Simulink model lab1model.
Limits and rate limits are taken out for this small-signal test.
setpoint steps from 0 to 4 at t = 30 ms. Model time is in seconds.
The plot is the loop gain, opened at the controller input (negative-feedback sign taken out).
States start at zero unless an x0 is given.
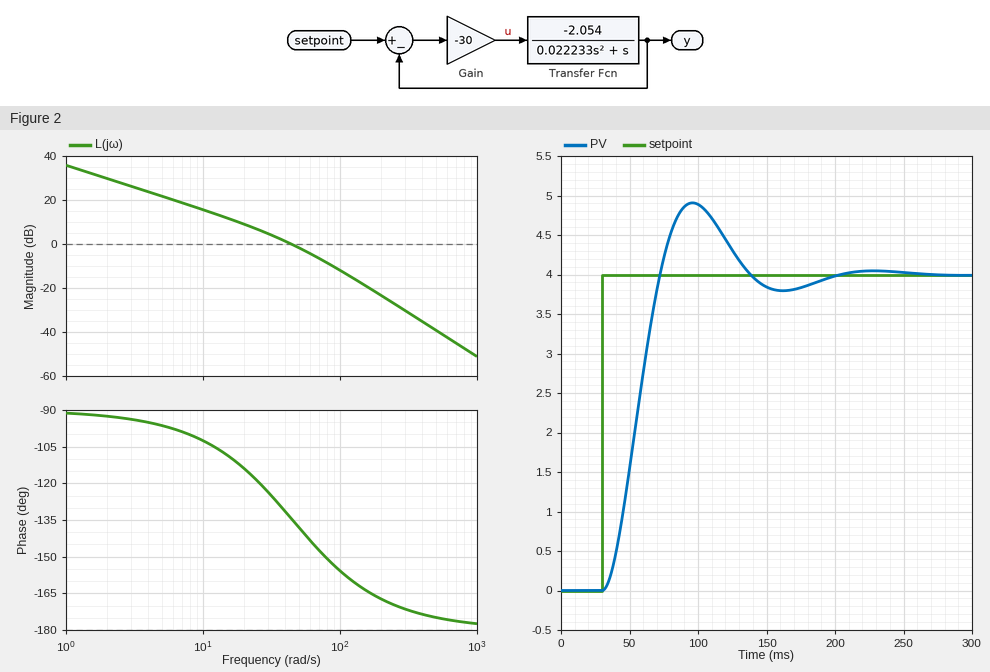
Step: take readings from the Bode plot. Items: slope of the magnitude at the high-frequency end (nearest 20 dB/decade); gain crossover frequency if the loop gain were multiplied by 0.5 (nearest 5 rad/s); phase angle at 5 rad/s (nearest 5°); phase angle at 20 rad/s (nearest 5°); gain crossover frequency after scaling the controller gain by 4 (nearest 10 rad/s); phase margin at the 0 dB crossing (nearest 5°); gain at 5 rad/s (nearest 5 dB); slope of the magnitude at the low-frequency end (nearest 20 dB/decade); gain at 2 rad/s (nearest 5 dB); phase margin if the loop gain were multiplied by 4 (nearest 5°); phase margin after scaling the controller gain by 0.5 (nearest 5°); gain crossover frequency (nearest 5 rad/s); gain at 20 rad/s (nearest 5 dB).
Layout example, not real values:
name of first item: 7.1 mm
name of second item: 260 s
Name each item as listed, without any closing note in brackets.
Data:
slope of the magnitude at the high-frequency end: -40 dB/decade
gain crossover frequency if the loop gain were multiplied by 0.5: 25 rad/s
phase angle at 5 rad/s: -95°
phase angle at 20 rad/s: -115°
gain crossover frequency after scaling the controller gain by 4: 100 rad/s
phase margin at the 0 dB crossing: 45°
gain at 5 rad/s: 20 dB
slope of the magnitude at the low-frequency end: -20 dB/decade
gain at 2 rad/s: 30 dB
phase margin if the loop gain were multiplied by 4: 25°
phase margin after scaling the controller gain by 0.5: 60°
gain crossover frequency: 45 rad/s
gain at 20 rad/s: 10 dB
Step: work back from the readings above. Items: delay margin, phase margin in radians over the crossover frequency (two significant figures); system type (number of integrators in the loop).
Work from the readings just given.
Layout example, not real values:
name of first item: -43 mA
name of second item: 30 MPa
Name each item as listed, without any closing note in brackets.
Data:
delay margin, phase margin in radians over the crossover frequency: 0.017 s
system type: 1
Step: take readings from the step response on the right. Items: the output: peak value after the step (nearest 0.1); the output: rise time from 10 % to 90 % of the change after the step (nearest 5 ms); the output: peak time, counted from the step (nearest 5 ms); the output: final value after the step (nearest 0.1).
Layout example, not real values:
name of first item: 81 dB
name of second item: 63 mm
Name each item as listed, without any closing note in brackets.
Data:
the output: peak value after the step: 4.9
the output: rise time from 10 % to 90 % of the change after the step: 30 ms
the output: peak time, counted from the step: 65 ms
the output: final value after the step: 4.0
